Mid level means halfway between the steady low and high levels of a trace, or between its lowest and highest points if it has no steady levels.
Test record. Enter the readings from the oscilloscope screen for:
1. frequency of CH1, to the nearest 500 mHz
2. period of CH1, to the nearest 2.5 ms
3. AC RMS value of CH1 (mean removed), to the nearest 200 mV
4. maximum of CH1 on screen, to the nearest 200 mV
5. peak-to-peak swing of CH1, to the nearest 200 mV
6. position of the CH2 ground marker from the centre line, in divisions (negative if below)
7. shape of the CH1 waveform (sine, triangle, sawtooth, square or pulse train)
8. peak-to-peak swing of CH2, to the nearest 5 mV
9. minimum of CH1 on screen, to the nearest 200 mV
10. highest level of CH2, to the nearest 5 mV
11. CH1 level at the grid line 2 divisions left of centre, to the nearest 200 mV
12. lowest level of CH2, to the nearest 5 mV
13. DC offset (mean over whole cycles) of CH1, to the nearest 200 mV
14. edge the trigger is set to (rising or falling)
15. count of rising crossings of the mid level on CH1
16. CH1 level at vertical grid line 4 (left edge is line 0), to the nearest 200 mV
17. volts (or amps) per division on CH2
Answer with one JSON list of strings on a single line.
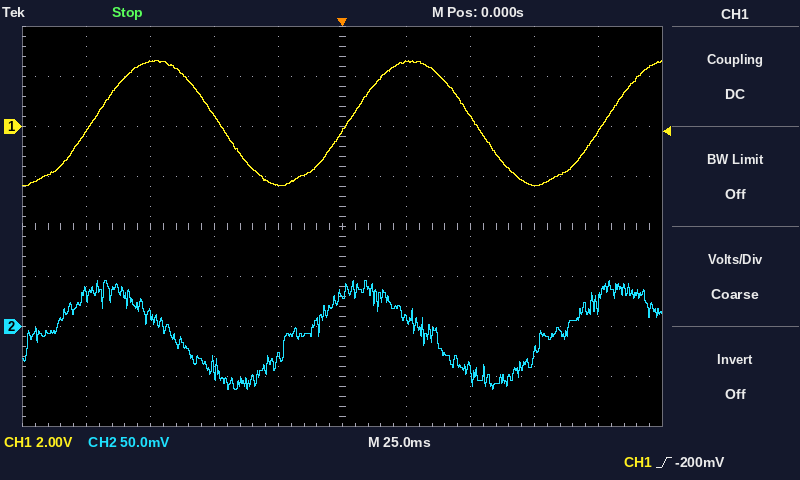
["10.0 Hz", "100.0 ms", "1.8 V", "2.6 V", "5.0 V", "-2.0 div", "sine", "110 mV", "-2.4 V", "45 mV", "400 mV", "-65 mV", "200 mV", "rising", "3", "-2.4 V", "50 mV"]
